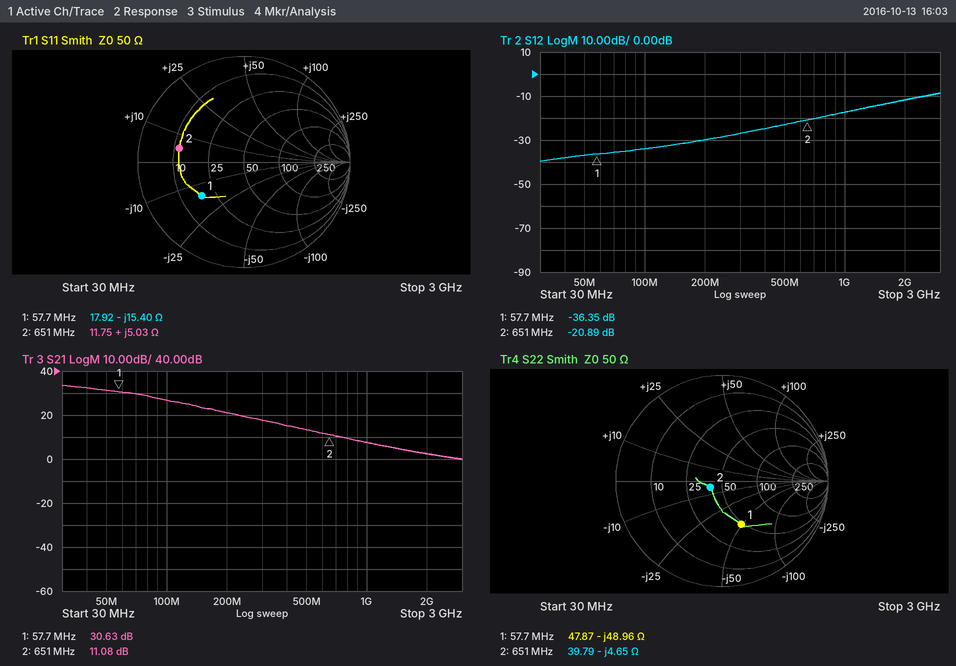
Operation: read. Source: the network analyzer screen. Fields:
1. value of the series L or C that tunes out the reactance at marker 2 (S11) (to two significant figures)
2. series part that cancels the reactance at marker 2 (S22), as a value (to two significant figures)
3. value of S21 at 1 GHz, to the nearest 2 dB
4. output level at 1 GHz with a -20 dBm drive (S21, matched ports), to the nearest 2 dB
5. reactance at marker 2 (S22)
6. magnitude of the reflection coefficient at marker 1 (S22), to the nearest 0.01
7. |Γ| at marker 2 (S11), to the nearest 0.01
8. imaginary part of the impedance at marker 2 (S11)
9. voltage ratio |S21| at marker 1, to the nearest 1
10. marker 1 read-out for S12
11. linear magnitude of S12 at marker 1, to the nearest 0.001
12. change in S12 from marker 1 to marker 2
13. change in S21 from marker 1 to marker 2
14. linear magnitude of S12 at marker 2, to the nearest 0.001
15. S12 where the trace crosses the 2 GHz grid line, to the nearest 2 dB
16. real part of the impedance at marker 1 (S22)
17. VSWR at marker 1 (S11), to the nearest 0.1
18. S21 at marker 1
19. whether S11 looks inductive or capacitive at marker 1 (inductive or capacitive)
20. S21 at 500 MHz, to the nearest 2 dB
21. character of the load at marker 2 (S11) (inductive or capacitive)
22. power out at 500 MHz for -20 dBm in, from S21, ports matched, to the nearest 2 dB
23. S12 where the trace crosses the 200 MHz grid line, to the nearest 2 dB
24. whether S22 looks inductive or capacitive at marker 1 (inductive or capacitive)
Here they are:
49 pF
1.1 nH
8 dB
-12 dBm
-4.65 Ω
0.45
0.62
+5.03 Ω
34
-36.35 dB
0.015
15.46 dB
-19.55 dB
0.090
-12 dB
47.87 Ω
3.1
30.63 dB
capacitive
14 dB
inductive
-6 dBm
-30 dB
capacitive
